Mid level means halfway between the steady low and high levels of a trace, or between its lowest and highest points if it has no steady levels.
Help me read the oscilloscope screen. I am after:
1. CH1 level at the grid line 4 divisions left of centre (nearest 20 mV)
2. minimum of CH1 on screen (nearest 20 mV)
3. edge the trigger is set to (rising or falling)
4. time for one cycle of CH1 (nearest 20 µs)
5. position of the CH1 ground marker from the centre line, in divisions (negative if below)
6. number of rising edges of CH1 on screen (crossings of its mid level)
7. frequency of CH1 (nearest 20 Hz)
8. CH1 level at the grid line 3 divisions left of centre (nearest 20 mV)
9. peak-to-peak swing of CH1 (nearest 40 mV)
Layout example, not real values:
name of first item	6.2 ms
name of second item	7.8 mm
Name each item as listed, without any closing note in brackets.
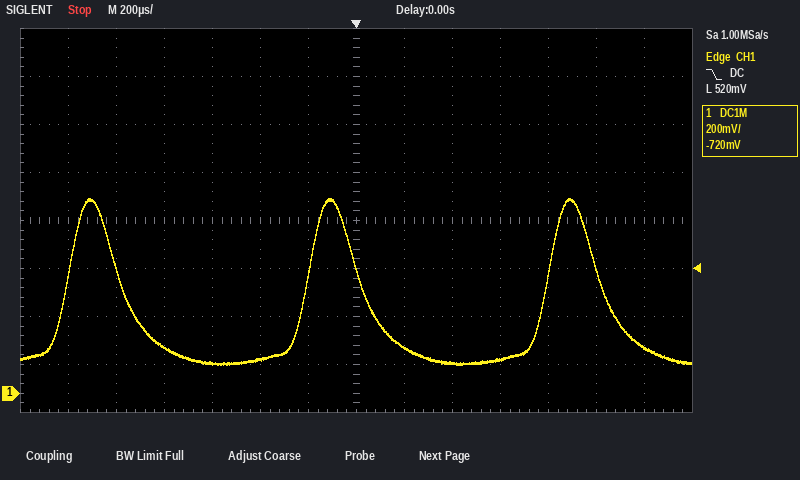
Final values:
CH1 level at the grid line 4 divisions left of centre	200 mV
minimum of CH1 on screen	120 mV
edge the trigger is set to	falling
time for one cycle of CH1	1.00 ms
position of the CH1 ground marker from the centre line, in divisions	-3.6 div
number of rising edges of CH1 on screen	3
frequency of CH1	1.00 kHz
CH1 level at the grid line 3 divisions left of centre	120 mV
peak-to-peak swing of CH1	680 mV
